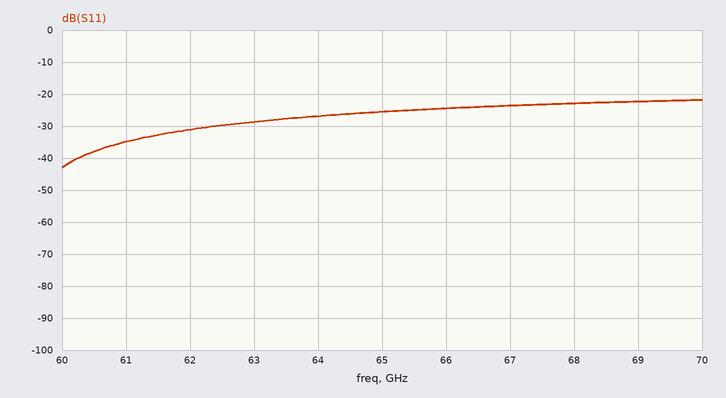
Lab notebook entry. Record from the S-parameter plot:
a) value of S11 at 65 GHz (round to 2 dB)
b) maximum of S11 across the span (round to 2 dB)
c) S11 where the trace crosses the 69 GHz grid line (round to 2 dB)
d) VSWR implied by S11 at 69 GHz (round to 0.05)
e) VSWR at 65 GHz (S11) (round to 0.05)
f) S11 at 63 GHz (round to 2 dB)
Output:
-26 dB
-22 dB
-22 dB
1.15
1.10
-28 dB
